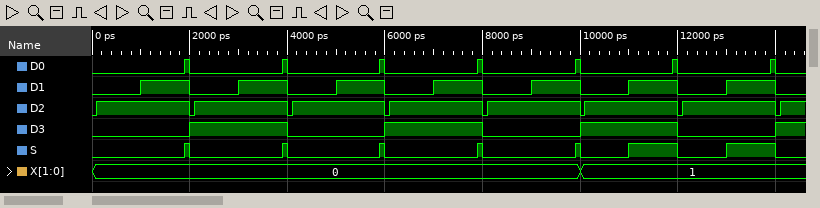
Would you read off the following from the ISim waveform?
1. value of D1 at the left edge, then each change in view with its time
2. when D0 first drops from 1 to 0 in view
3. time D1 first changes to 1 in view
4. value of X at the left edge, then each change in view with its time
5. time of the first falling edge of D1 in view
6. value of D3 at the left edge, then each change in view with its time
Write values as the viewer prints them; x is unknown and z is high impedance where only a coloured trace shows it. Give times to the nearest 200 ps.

0, 1 at 1000 ps, 0 at 2000 ps, 1 at 3000 ps, 0 at 4000 ps, 1 at 5000 ps, 0 at 6000 ps, 1 at 7000 ps, 0 at 8000 ps, 1 at 9000 ps, 0 at 10000 ps, 1 at 11000 ps, 0 at 12000 ps, 1 at 13000 ps, 0 at 14000 ps
2000 ps
1000 ps
0, 1 at 10000 ps
2000 ps
0, 1 at 2000 ps, 0 at 4000 ps, 1 at 6000 ps, 0 at 8000 ps, 1 at 10000 ps, 0 at 12000 ps, 1 at 14000 ps
